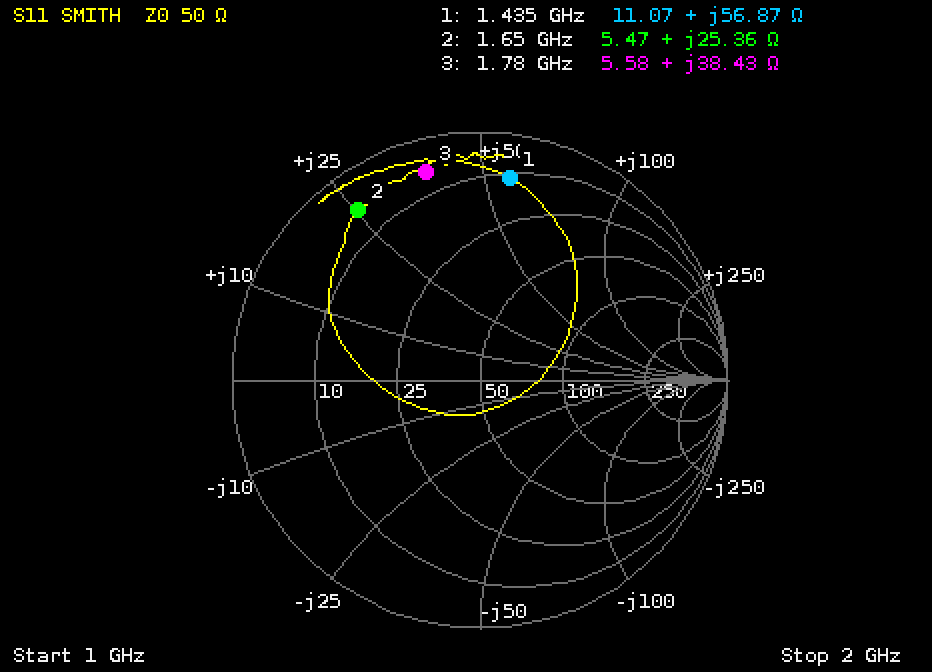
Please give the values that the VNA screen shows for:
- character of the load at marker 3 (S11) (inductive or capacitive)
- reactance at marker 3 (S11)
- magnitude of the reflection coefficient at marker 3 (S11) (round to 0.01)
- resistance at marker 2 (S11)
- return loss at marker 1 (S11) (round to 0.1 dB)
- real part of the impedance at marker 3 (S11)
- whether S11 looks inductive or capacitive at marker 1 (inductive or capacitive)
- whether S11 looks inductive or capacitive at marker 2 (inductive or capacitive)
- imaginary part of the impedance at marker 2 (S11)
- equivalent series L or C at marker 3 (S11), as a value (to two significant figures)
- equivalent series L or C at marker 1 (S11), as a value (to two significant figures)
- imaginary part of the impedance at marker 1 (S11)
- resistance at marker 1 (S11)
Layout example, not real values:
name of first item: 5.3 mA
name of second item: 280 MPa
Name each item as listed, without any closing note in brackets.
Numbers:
character of the load at marker 3 (S11): inductive
reactance at marker 3: +38.43 Ω
magnitude of the reflection coefficient at marker 3 (S11): 0.87
resistance at marker 2: 5.47 Ω
return loss at marker 1 (S11): 1.7 dB
real part of the impedance at marker 3: 5.58 Ω
whether S11 looks inductive or capacitive at marker 1: inductive
whether S11 looks inductive or capacitive at marker 2: inductive
imaginary part of the impedance at marker 2: +25.36 Ω
equivalent series L or C at marker 3 (S11), as a value: 3.4 nH
equivalent series L or C at marker 1 (S11), as a value: 6.3 nH
imaginary part of the impedance at marker 1: +56.87 Ω
resistance at marker 1: 11.07 Ω
